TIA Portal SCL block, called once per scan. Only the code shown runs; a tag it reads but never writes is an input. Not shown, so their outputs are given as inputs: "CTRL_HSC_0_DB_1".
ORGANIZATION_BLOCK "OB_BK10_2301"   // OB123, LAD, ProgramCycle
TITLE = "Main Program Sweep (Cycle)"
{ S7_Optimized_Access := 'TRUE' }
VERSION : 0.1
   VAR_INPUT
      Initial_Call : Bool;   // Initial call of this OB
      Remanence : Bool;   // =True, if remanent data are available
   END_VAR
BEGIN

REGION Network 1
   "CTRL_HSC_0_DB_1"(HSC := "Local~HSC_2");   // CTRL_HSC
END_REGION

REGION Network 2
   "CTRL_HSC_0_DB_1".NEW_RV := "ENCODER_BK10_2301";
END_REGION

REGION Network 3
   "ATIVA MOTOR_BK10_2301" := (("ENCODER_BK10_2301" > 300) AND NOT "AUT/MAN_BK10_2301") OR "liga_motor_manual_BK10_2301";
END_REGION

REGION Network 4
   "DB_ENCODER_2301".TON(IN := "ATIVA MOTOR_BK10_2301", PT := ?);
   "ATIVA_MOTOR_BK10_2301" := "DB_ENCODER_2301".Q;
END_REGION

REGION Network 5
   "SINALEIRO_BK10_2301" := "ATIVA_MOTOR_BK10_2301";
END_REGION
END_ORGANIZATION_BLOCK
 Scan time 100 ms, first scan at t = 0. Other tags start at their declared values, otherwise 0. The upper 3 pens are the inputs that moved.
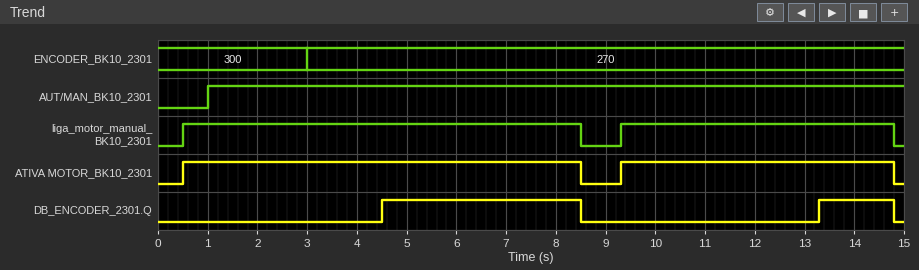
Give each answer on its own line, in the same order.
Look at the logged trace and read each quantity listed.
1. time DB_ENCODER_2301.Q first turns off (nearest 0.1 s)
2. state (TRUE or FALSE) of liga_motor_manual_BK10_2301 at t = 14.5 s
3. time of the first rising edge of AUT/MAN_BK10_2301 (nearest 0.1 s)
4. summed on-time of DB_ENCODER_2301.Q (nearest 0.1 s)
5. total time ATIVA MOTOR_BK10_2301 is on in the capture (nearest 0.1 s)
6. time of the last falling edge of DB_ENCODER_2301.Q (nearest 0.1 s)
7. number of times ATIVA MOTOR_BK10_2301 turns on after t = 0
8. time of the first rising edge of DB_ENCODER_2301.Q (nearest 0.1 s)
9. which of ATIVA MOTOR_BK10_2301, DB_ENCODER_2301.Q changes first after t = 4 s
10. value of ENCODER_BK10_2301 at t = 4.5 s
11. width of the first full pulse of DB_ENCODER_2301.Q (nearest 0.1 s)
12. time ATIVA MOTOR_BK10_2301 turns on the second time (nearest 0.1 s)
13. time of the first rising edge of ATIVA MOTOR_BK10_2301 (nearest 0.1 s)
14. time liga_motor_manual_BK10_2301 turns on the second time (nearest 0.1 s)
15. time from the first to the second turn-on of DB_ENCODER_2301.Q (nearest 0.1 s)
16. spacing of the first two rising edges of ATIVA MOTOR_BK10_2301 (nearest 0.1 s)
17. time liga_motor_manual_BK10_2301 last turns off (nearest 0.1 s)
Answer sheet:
8.5 s
TRUE
1.0 s
5.5 s
13.5 s
14.8 s
2
4.5 s
DB_ENCODER_2301.Q
270
4.0 s
9.3 s
0.5 s
9.3 s
8.8 s
8.8 s
14.8 s
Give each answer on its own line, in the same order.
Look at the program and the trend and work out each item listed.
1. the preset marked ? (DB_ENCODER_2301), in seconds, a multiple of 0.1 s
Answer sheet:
4.0 s
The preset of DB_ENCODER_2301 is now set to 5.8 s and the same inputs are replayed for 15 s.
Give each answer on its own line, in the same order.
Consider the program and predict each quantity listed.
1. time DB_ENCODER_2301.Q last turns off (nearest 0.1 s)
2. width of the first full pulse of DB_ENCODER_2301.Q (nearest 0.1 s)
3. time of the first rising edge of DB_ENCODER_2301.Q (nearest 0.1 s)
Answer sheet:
8.5 s
2.2 s
6.3 s
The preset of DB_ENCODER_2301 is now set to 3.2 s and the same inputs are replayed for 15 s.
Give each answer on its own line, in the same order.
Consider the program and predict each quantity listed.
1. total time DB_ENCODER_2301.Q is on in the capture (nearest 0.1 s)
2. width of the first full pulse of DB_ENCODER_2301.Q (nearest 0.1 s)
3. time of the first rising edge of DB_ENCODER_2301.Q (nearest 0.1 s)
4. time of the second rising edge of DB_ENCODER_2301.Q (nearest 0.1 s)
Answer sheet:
7.1 s
4.8 s
3.7 s
12.5 s
